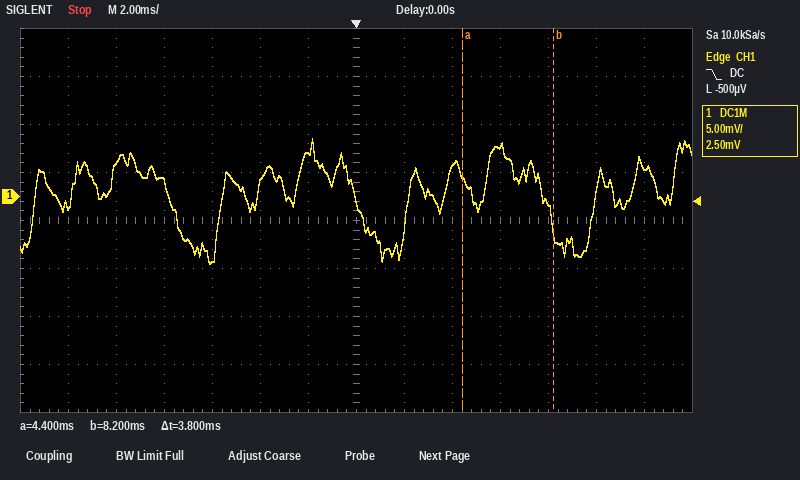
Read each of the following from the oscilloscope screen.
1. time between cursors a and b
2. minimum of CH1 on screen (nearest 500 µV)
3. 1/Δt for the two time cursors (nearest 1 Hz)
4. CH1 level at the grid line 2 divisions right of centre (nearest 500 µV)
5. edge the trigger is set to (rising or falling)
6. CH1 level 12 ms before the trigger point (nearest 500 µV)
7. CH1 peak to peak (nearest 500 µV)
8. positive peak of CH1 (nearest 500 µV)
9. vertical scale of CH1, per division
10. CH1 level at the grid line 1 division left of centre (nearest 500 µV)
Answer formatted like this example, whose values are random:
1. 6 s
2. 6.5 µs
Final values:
1. 3.8 ms
2. -7.0 mV
3. 263 Hz
4. 3.0 mV
5. falling
6. -1.0 mV
7. 13.0 mV
8. 6.0 mV
9. 5 mV
10. 4.5 mV
